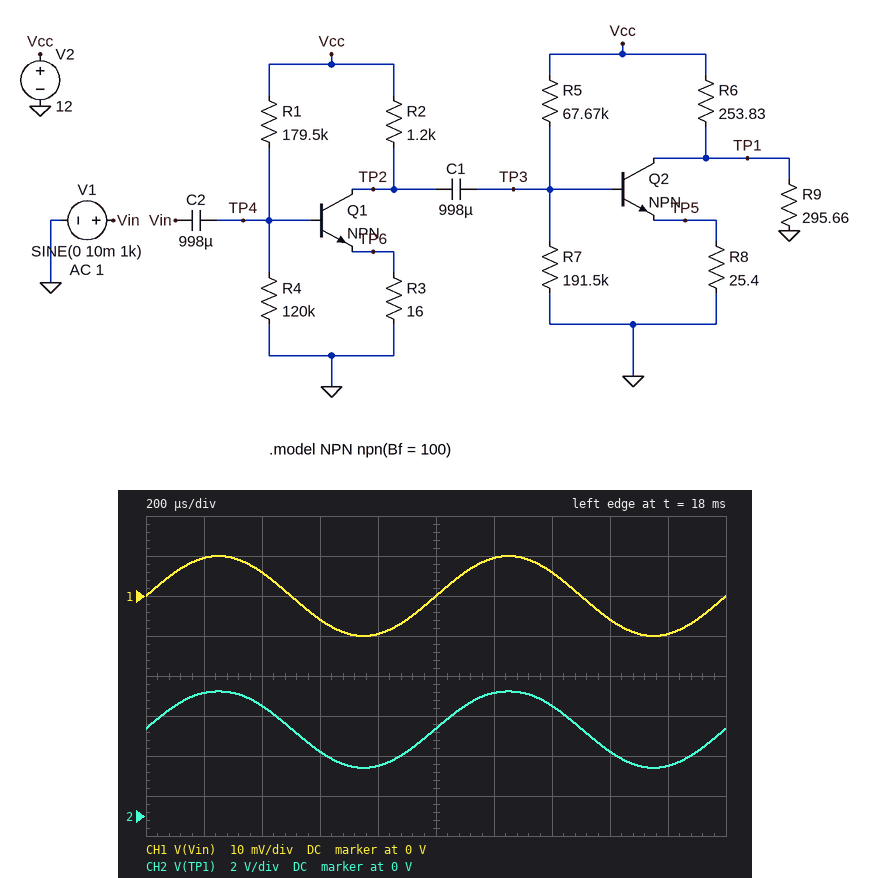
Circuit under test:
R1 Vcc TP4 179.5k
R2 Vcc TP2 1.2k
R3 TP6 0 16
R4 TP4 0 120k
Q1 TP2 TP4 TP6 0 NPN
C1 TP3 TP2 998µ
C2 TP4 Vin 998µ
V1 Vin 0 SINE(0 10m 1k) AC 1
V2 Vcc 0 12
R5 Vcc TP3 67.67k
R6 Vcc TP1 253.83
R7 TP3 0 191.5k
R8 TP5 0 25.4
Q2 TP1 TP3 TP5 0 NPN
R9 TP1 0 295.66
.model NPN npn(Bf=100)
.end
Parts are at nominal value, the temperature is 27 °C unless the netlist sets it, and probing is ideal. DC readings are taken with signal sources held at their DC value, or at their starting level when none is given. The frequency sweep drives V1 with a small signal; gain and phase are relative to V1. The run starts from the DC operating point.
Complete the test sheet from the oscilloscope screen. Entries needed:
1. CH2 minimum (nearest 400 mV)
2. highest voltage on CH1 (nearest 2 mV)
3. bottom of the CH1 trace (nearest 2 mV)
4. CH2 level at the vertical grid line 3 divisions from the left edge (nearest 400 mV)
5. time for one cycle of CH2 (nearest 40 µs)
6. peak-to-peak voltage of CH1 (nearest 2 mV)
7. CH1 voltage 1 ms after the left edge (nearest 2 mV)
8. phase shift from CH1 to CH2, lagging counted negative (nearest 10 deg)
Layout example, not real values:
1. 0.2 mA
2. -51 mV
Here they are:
1. 2.4 V
2. 10 mV
3. -10 mV
4. 3.2 V
5. 1.00 ms
6. 20 mV
7. 0 V
8. 0 deg
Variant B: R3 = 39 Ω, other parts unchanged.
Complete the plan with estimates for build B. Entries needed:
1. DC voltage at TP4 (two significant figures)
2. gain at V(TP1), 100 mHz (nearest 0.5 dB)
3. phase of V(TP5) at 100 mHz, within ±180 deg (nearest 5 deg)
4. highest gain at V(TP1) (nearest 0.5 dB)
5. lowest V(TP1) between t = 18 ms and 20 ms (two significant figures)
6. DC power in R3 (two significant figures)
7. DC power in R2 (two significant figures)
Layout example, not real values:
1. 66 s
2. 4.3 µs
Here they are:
1. 1.0 V
2. 38.0 dB
3. -135 deg
4. 39.5 dB
5. 3.4 V
6. 1.1 mW
7. 33 mW
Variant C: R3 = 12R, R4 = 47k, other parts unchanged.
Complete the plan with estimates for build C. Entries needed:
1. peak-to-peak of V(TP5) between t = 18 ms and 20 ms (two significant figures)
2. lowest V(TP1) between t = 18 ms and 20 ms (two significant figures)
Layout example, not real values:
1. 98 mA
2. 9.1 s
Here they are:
1. 810 mV
2. 2.1 V
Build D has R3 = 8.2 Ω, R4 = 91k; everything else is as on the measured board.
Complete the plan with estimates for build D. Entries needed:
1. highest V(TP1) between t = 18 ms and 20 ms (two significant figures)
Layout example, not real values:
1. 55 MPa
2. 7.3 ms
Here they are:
1. 6.5 V
